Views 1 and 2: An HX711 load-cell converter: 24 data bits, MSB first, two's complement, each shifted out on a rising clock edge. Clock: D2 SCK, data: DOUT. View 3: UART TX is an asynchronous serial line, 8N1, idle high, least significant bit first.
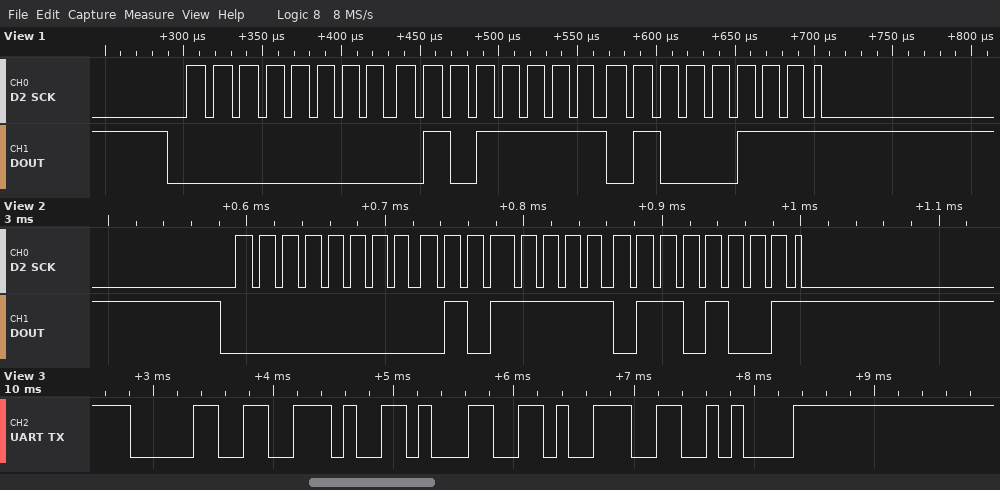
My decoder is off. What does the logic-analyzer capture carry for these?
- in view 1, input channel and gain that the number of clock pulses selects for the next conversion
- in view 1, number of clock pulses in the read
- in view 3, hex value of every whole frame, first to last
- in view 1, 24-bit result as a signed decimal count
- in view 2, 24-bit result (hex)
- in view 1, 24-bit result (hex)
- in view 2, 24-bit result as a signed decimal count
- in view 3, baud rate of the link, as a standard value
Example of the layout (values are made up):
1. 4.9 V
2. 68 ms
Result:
1. channel A, gain 128
2. 25
3. 30 2E 31 39 0A
4. 24391
5. 0x005F69
6. 0x005F47
7. 24425
8. 9600 baud
